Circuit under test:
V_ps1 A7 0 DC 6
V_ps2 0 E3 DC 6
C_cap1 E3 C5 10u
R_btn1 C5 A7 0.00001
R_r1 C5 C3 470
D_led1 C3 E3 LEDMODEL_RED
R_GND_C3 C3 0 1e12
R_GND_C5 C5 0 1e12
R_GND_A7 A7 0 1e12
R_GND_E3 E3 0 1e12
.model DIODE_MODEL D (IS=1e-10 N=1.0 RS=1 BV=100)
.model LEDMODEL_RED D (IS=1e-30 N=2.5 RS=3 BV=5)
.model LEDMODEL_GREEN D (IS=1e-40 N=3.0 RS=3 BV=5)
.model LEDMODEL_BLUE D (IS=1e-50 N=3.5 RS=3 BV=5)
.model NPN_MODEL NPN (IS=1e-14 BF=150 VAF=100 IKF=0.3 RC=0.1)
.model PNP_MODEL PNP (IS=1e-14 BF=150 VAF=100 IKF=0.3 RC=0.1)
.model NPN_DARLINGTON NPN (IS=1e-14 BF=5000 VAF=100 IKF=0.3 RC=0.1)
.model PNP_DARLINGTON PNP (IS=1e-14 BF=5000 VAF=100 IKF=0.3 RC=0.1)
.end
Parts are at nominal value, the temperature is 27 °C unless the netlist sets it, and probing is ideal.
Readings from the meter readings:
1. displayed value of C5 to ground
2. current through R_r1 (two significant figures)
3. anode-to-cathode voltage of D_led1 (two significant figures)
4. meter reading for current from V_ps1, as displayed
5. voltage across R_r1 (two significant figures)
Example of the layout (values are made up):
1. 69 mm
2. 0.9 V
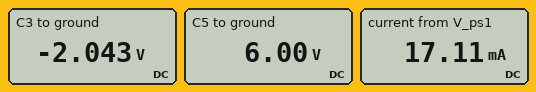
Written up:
1. 6.00 V
2. 17 mA
3. 4.0 V
4. 17.11 mA
5. 8.0 V
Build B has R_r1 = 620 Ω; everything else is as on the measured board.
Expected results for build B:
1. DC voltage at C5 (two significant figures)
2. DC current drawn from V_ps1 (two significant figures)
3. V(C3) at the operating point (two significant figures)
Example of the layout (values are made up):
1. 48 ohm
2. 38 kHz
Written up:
1. 6.0 V
2. 13 mA
3. -2.1 V
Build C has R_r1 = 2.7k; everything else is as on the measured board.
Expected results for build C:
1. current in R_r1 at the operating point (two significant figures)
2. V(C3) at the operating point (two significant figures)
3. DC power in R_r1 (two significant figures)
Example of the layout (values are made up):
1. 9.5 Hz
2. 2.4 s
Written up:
1. 3.0 mA
2. -2.2 V
3. 25 mW
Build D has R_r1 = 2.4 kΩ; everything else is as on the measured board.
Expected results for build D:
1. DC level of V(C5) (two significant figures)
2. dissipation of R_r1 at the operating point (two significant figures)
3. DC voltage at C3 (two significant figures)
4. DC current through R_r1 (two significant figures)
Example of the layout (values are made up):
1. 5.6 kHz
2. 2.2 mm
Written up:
1. 6.0 V
2. 28 mW
3. -2.2 V
4. 3.4 mA
